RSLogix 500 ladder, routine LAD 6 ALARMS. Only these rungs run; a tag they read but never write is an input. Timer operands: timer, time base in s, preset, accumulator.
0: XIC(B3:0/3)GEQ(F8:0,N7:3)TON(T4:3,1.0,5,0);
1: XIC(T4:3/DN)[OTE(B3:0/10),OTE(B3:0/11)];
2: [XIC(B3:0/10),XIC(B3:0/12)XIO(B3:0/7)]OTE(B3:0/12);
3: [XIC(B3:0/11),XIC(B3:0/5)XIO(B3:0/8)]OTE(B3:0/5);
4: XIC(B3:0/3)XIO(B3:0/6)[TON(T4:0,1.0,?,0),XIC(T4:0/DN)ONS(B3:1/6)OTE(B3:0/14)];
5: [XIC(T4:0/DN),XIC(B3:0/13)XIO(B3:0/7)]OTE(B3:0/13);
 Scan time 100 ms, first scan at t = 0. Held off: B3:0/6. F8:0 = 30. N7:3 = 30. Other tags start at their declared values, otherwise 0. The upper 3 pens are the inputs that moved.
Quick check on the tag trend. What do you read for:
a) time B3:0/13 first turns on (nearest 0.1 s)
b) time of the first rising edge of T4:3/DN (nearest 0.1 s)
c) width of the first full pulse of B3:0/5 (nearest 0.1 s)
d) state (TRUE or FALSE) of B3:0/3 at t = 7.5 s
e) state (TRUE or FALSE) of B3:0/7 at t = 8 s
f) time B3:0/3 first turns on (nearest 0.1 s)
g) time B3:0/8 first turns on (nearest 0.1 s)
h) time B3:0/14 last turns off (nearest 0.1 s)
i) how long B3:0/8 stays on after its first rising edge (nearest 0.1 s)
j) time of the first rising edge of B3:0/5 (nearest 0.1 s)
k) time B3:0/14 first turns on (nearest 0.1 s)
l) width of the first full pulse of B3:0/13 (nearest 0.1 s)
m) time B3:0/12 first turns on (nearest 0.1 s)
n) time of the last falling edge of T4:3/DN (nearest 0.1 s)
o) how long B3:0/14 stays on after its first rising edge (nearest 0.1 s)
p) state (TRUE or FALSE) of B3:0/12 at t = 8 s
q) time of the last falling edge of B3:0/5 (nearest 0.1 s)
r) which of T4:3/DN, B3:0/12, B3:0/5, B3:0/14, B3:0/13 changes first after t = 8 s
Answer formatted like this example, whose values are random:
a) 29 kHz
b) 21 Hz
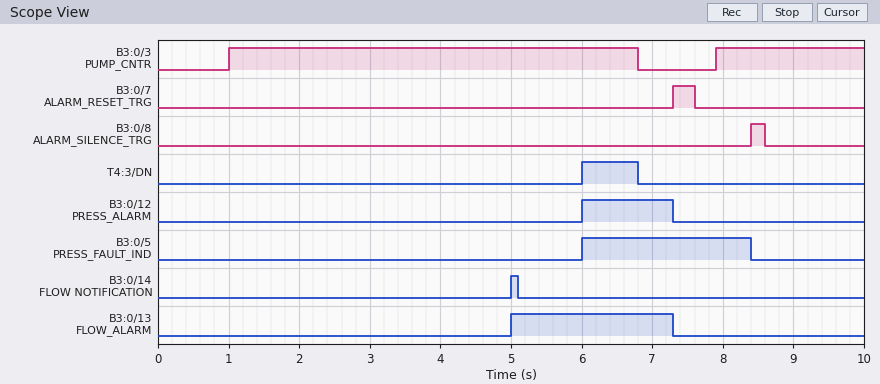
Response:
a) 5.0 s
b) 6.0 s
c) 2.4 s
d) FALSE
e) FALSE
f) 1.0 s
g) 8.4 s
h) 5.1 s
i) 0.2 s
j) 6.0 s
k) 5.0 s
l) 2.3 s
m) 6.0 s
n) 6.8 s
o) 0.1 s
p) FALSE
q) 8.4 s
r) B3:0/5
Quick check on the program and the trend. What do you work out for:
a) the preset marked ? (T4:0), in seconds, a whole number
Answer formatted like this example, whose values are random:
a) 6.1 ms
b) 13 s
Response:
a) 4 s
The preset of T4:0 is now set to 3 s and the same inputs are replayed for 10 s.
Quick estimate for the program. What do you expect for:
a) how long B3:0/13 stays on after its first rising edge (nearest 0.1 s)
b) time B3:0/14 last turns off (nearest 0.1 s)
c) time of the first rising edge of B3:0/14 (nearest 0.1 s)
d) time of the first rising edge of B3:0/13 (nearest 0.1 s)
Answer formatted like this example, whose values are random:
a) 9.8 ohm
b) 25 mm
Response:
a) 3.3 s
b) 4.1 s
c) 4.0 s
d) 4.0 s
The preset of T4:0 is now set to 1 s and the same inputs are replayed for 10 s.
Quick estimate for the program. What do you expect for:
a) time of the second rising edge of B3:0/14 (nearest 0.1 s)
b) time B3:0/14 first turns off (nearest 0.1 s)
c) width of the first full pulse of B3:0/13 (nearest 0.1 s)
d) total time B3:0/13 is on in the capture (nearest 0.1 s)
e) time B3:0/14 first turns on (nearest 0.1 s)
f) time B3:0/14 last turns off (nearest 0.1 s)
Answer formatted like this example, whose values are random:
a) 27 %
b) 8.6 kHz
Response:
a) 8.9 s
b) 2.1 s
c) 5.3 s
d) 6.4 s
e) 2.0 s
f) 9.0 s
